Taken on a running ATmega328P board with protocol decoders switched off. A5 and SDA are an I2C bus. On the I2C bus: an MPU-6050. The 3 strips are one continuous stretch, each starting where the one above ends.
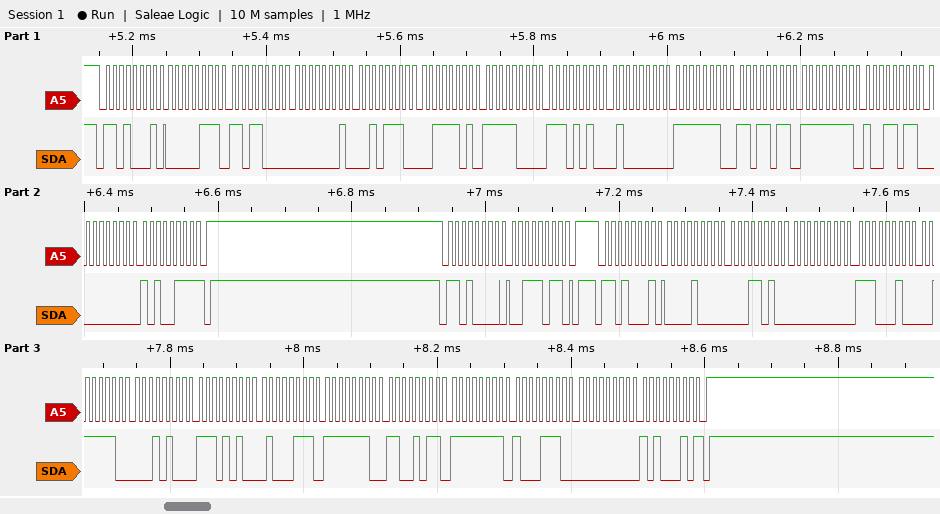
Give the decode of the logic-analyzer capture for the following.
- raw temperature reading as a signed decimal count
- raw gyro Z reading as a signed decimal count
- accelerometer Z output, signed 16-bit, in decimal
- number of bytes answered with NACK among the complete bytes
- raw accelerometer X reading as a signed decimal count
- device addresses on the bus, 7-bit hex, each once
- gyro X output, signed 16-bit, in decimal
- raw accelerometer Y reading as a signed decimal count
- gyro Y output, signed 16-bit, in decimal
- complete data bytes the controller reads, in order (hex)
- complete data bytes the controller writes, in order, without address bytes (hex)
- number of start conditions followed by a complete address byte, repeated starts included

-5561
162
15892
2
2074
0x68
-309
226
-114
07 D8 01 2E 3D F8 EA 40 FE DB FF 9B 00 A7 08 1A 00 E2 3E 14 EA 47 FE CB FF 8E 00 A2
3B
3
